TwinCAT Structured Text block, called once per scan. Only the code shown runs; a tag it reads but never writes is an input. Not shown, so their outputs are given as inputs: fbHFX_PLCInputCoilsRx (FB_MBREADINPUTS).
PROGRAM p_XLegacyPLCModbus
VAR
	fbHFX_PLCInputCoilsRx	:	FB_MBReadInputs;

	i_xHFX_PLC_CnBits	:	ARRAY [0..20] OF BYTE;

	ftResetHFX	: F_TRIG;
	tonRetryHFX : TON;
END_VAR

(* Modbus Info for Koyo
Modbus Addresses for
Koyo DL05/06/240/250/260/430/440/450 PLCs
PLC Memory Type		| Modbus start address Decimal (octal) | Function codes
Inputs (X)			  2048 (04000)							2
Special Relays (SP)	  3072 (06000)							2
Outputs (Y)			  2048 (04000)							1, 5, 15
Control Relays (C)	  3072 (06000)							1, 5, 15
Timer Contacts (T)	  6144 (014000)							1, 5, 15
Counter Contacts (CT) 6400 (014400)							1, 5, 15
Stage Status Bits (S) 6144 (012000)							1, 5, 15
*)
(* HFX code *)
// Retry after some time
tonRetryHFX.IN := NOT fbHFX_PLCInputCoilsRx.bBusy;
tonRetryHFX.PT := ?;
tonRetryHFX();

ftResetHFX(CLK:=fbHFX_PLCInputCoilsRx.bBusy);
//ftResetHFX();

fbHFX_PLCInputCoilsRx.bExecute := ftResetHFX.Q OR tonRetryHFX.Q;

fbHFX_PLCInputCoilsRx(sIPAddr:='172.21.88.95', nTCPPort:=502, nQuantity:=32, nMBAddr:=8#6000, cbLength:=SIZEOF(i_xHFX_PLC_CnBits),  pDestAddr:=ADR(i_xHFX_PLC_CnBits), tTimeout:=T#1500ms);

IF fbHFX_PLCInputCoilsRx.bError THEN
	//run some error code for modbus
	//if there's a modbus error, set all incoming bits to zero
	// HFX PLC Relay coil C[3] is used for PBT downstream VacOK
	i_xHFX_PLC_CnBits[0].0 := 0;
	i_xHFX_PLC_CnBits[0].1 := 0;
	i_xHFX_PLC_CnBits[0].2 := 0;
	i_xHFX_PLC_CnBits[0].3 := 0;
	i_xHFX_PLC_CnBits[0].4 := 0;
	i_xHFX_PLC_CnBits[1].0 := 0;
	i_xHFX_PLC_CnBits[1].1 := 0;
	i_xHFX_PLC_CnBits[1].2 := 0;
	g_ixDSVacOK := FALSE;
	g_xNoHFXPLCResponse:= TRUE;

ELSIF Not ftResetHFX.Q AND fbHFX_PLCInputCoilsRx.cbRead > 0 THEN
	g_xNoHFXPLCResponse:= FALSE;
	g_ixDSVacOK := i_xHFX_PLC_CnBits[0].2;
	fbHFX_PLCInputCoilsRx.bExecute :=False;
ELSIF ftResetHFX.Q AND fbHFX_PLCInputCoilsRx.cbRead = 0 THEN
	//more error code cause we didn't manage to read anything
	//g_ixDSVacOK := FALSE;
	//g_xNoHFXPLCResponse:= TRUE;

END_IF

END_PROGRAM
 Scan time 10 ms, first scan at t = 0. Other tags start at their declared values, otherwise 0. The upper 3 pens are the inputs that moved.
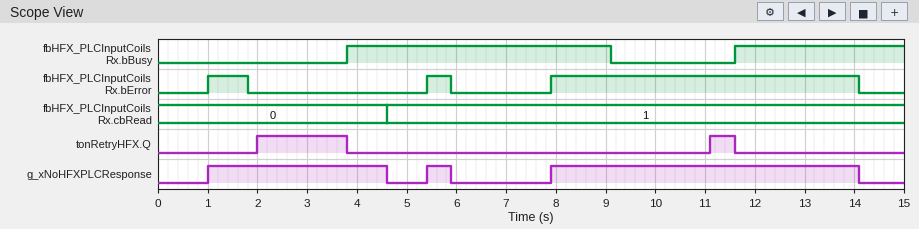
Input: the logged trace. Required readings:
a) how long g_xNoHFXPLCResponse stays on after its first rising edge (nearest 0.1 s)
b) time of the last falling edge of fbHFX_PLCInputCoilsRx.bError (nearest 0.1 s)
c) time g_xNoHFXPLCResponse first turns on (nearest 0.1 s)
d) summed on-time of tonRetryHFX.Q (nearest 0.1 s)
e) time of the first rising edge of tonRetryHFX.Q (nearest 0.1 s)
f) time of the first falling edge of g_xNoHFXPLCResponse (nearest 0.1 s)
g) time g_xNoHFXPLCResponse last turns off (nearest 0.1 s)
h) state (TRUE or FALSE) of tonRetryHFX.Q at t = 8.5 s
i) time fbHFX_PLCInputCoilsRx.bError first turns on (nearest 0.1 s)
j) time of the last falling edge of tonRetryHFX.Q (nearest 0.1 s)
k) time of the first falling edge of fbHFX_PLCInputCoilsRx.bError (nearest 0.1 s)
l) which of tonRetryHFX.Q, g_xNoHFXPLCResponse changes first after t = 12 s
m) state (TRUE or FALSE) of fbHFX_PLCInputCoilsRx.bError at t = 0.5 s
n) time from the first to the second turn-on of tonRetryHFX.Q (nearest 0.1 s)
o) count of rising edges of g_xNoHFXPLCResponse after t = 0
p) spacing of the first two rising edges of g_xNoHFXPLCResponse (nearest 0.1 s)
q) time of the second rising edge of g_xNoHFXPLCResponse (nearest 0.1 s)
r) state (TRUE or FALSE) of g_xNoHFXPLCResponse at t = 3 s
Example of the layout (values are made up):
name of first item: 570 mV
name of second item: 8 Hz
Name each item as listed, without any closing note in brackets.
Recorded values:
how long g_xNoHFXPLCResponse stays on after its first rising edge: 3.6 s
time of the last falling edge of fbHFX_PLCInputCoilsRx.bError: 14.1 s
time g_xNoHFXPLCResponse first turns on: 1.0 s
summed on-time of tonRetryHFX.Q: 2.3 s
time of the first rising edge of tonRetryHFX.Q: 2.0 s
time of the first falling edge of g_xNoHFXPLCResponse: 4.6 s
time g_xNoHFXPLCResponse last turns off: 14.1 s
state (TRUE or FALSE) of tonRetryHFX.Q at t = 8.5 s: FALSE
time fbHFX_PLCInputCoilsRx.bError first turns on: 1.0 s
time of the last falling edge of tonRetryHFX.Q: 11.6 s
time of the first falling edge of fbHFX_PLCInputCoilsRx.bError: 1.8 s
which of tonRetryHFX.Q, g_xNoHFXPLCResponse changes first after t = 12 s: g_xNoHFXPLCResponse
state (TRUE or FALSE) of fbHFX_PLCInputCoilsRx.bError at t = 0.5 s: FALSE
time from the first to the second turn-on of tonRetryHFX.Q: 9.1 s
count of rising edges of g_xNoHFXPLCResponse after t = 0: 3
spacing of the first two rising edges of g_xNoHFXPLCResponse: 4.4 s
time of the second rising edge of g_xNoHFXPLCResponse: 5.4 s
state (TRUE or FALSE) of g_xNoHFXPLCResponse at t = 3 s: TRUE
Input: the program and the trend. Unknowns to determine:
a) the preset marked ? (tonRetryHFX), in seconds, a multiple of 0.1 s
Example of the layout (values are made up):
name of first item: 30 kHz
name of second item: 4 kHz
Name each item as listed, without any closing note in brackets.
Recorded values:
the preset marked ? (tonRetryHFX), in seconds, a multiple of 0.1 s: 2.0 s
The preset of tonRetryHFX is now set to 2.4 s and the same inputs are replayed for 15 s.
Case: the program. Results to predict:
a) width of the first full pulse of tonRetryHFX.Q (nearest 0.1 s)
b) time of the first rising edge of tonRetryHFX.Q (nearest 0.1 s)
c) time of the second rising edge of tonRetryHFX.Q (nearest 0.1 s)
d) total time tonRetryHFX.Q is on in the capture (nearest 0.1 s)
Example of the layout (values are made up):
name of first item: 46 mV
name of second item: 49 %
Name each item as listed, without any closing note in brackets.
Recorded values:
width of the first full pulse of tonRetryHFX.Q: 1.4 s
time of the first rising edge of tonRetryHFX.Q: 2.4 s
time of the second rising edge of tonRetryHFX.Q: 11.5 s
total time tonRetryHFX.Q is on in the capture: 1.5 s
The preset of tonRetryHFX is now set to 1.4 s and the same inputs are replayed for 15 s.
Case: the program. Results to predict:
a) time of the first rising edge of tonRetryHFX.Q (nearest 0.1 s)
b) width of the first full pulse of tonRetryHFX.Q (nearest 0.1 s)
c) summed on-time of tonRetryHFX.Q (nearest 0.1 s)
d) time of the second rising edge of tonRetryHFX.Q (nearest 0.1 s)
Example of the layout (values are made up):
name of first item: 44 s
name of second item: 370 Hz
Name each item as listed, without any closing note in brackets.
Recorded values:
time of the first rising edge of tonRetryHFX.Q: 1.4 s
width of the first full pulse of tonRetryHFX.Q: 2.4 s
summed on-time of tonRetryHFX.Q: 3.5 s
time of the second rising edge of tonRetryHFX.Q: 10.5 s
